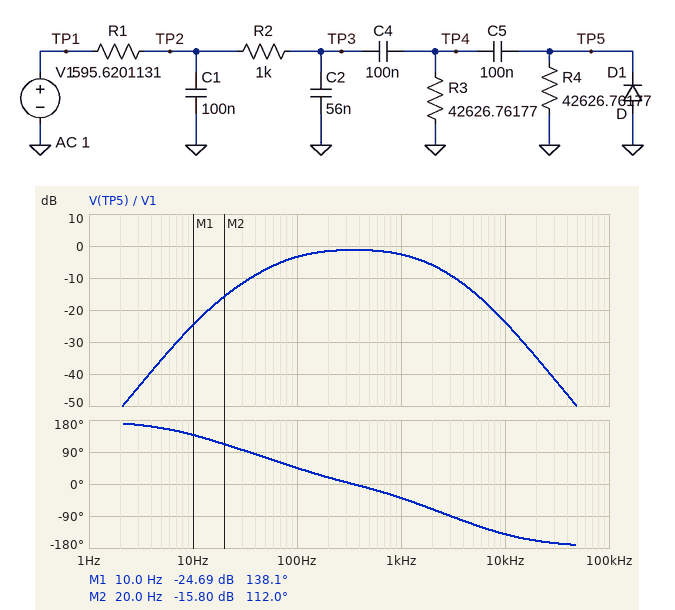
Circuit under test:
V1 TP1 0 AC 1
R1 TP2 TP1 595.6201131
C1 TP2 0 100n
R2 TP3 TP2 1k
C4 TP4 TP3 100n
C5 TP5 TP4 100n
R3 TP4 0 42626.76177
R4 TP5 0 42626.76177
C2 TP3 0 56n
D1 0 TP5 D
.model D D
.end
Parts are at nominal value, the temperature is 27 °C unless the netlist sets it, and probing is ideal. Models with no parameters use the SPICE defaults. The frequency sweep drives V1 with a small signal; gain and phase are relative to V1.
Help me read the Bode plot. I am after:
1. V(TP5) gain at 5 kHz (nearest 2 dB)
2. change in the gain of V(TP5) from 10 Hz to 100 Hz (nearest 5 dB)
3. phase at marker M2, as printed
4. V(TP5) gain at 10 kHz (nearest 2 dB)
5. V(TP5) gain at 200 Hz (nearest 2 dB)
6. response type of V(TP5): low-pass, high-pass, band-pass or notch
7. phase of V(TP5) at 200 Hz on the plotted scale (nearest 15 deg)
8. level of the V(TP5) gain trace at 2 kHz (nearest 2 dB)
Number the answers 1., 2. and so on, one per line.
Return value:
1. -14 dB
2. 20 dB
3. 112.0 deg
4. -24 dB
5. -2 dB
6. band-pass
7. 15 deg
8. -6 dB
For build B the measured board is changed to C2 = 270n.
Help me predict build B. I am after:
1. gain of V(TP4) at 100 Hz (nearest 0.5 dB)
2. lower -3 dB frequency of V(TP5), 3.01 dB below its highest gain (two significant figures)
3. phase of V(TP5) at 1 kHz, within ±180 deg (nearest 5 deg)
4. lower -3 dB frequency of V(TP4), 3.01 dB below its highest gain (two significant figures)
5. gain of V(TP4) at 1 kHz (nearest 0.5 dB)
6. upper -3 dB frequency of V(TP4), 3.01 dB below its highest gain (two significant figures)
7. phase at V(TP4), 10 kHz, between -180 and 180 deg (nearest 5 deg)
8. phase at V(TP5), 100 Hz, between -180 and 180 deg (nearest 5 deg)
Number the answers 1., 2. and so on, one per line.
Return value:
1. -3.0 dB
2. 66 Hz
3. -75 deg
4. 50 Hz
5. -10.0 dB
6. 520 Hz
7. -155 deg
8. 35 deg
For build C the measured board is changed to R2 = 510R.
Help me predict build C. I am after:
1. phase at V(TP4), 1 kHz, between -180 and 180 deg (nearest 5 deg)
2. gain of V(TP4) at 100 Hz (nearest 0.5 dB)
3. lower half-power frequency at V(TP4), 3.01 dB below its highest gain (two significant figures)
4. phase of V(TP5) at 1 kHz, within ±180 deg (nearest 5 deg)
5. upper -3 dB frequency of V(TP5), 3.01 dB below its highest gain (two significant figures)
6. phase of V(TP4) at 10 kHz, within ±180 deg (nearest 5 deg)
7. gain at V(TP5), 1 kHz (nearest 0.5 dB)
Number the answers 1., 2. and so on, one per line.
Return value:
1. -35 deg
2. -2.5 dB
3. 71 Hz
4. -30 deg
5. 1.7 kHz
6. -125 deg
7. -2.0 dB
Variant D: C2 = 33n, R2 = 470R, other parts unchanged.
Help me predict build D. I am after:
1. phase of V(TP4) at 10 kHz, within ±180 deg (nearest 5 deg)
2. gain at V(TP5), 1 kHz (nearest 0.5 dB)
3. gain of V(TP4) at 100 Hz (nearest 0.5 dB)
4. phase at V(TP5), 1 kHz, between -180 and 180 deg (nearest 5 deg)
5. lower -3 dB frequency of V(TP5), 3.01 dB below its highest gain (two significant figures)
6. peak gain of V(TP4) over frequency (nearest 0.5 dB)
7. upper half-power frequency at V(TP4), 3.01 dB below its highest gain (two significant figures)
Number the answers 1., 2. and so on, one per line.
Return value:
1. -115 deg
2. -1.5 dB
3. -2.5 dB
4. -25 deg
5. 87 Hz
6. -1.0 dB
7. 2.1 kHz
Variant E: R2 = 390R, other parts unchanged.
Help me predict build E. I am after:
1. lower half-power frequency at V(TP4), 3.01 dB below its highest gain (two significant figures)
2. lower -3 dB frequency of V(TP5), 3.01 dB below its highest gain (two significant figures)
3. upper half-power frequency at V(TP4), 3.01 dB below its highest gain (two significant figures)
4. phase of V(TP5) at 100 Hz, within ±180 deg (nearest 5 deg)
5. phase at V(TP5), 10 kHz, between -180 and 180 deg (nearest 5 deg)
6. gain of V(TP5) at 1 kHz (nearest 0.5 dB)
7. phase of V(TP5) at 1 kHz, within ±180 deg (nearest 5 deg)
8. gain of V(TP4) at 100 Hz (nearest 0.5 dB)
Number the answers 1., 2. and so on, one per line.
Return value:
1. 71 Hz
2. 86 Hz
3. 1.8 kHz
4. 45 deg
5. -120 deg
6. -2.0 dB
7. -30 deg
8. -2.5 dB
